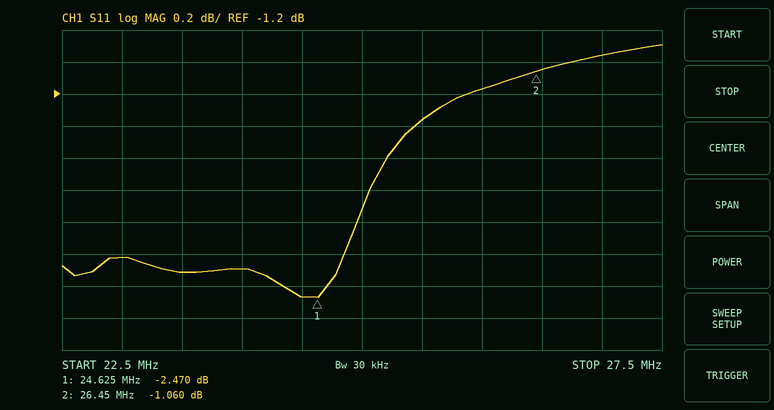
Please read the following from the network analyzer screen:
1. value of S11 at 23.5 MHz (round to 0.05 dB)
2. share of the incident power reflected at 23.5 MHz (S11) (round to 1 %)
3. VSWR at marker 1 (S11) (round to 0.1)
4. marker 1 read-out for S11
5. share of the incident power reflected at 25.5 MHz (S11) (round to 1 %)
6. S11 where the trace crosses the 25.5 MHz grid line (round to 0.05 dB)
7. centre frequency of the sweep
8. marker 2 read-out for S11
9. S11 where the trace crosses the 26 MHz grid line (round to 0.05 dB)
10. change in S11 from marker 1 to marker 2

-2.30 dB
59 %
7.1
-2.470 dB
73 %
-1.35 dB
25 MHz
-1.060 dB
-1.15 dB
1.410 dB
